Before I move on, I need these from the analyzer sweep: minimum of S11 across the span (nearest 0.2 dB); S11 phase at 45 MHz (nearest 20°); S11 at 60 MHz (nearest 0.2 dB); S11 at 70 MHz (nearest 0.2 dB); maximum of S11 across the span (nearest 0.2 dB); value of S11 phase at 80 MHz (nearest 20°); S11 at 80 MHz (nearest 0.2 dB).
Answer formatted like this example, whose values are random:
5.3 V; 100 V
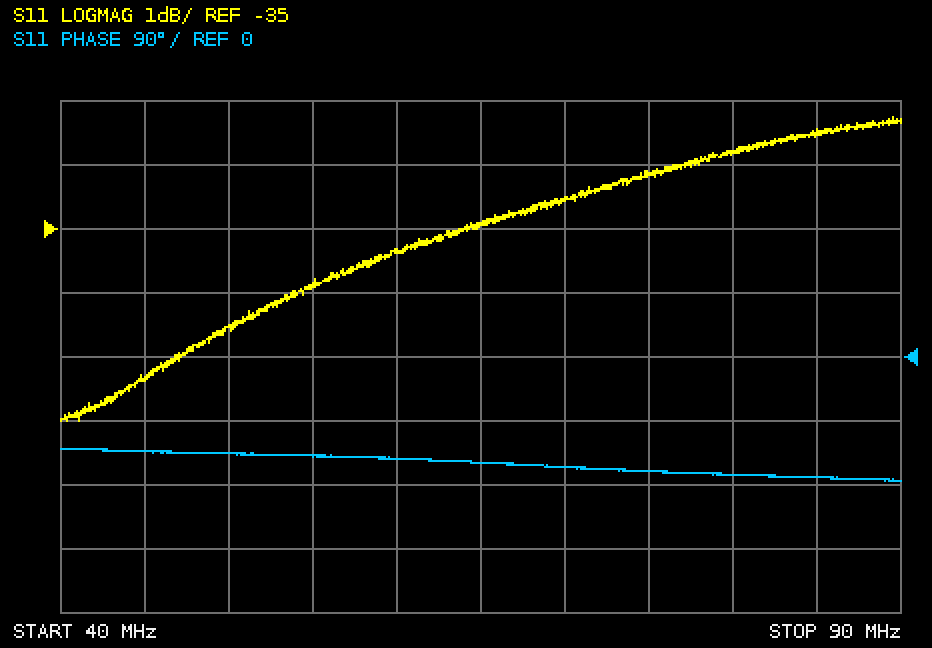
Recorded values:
-38.0 dB; -140°; -35.4 dB; -34.6 dB; -33.2 dB; -160°; -33.8 dB
